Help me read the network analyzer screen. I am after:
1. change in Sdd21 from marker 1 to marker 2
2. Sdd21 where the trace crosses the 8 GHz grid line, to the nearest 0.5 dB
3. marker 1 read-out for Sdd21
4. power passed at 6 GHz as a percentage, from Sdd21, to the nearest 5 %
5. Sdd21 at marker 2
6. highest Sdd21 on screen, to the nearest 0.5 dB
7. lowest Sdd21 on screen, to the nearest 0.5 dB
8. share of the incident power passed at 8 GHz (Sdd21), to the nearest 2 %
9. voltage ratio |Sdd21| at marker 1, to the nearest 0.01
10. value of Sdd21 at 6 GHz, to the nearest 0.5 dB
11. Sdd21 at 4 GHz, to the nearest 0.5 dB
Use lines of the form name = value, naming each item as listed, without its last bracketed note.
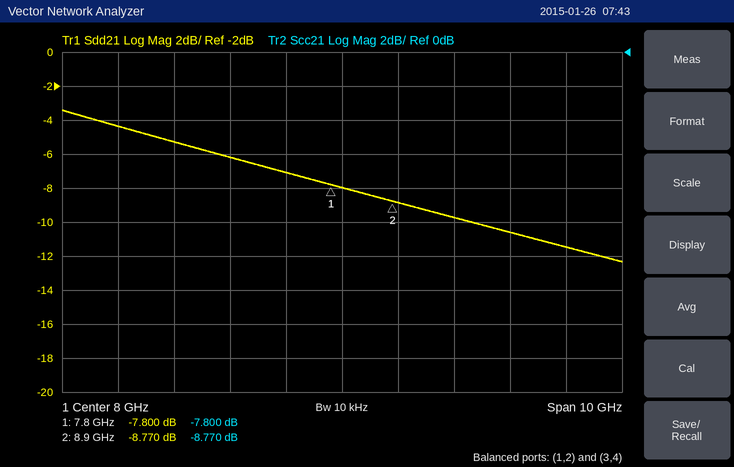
change in Sdd21 from marker 1 to marker 2 = -0.970 dB
Sdd21 where the trace crosses the 8 GHz grid line, to the nearest 0.5 dB = -8.0 dB
marker 1 read-out for Sdd21 = -7.800 dB
power passed at 6 GHz as a percentage, from Sdd21, to the nearest 5 % = 25 %
Sdd21 at marker 2 = -8.770 dB
highest Sdd21 on screen, to the nearest 0.5 dB = -3.5 dB
lowest Sdd21 on screen, to the nearest 0.5 dB = -12.5 dB
share of the incident power passed at 8 GHz (Sdd21), to the nearest 2 % = 16 %
voltage ratio |Sdd21| at marker 1, to the nearest 0.01 = 0.41
value of Sdd21 at 6 GHz, to the nearest 0.5 dB = -6.0 dB
Sdd21 at 4 GHz, to the nearest 0.5 dB = -4.5 dB
